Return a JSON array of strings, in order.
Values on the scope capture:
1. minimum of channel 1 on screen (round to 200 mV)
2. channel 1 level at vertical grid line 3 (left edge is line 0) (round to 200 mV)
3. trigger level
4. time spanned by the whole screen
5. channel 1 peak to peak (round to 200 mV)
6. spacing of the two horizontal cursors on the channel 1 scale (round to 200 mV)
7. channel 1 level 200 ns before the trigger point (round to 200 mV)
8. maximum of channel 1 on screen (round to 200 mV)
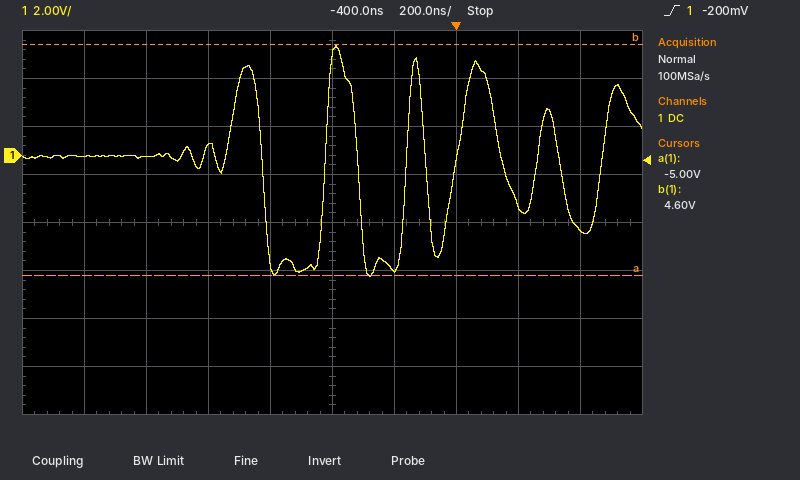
["-5.0 V", "400 mV", "-200 mV", "2 µs", "9.6 V", "9.6 V", "-4.8 V", "4.6 V"]
